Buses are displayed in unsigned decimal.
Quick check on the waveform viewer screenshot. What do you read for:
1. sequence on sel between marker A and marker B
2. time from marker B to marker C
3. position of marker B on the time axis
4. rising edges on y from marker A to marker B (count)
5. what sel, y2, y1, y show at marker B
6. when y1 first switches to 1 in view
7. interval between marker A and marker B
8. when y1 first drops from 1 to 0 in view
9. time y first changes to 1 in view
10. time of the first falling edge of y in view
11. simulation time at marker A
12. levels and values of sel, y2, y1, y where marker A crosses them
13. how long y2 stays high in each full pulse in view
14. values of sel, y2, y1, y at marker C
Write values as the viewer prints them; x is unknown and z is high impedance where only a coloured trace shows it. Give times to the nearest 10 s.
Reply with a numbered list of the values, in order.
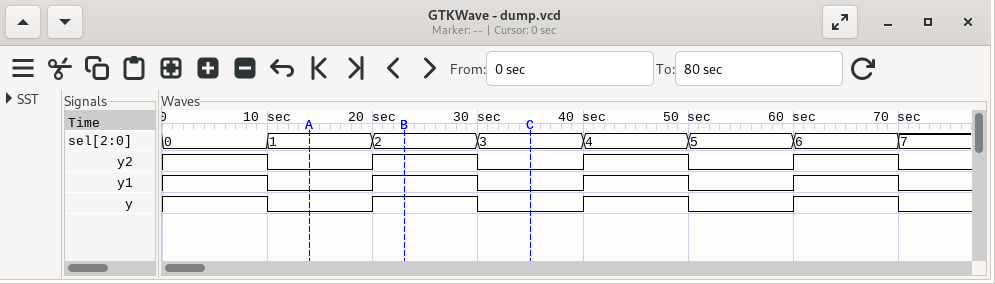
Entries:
1. 1, 2
2. 10 s
3. 20 s
4. 1
5. sel=2, y2=1, y1=1, y=1
6. 20 s
7. 10 s
8. 10 s
9. 20 s
10. 10 s
11. 10 s
12. sel=1, y2=0, y1=0, y=0
13. 10 s, 10 s, 10 s
14. sel=3, y2=0, y1=0, y=0
